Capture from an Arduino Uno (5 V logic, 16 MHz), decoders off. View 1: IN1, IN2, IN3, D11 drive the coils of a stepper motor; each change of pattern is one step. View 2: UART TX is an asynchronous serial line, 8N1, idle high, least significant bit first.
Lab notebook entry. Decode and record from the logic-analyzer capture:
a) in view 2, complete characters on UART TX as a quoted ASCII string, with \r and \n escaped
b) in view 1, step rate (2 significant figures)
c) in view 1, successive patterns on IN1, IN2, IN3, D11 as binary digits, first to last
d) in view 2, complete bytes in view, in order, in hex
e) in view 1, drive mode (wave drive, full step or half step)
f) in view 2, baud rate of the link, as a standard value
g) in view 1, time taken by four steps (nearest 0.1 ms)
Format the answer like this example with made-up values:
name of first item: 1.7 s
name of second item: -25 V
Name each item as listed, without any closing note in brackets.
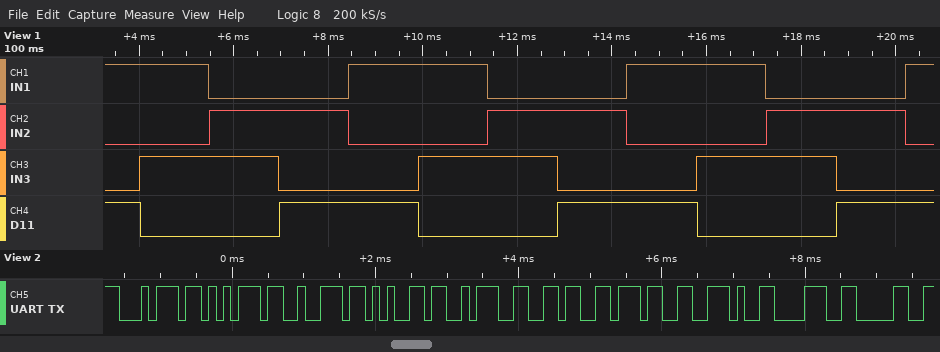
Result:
in view 2, complete characters on UART TX as a quoted ASCII string, with \r and \n escaped: "ture:67.80"
in view 1, step rate: 680 steps/s
in view 1, successive patterns on IN1, IN2, IN3, D11 as binary digits, first to last: 1001 1010 0110 0101 1001 1010 0110 0101 1001 1010 0110 0101 1001
in view 2, complete bytes in view, in order, in hex: 74 75 72 65 3A 36 37 2E 38 30
in view 1, drive mode: full step
in view 2, baud rate of the link, as a standard value: 9600 baud
in view 1, time taken by four steps: 5.9 ms
